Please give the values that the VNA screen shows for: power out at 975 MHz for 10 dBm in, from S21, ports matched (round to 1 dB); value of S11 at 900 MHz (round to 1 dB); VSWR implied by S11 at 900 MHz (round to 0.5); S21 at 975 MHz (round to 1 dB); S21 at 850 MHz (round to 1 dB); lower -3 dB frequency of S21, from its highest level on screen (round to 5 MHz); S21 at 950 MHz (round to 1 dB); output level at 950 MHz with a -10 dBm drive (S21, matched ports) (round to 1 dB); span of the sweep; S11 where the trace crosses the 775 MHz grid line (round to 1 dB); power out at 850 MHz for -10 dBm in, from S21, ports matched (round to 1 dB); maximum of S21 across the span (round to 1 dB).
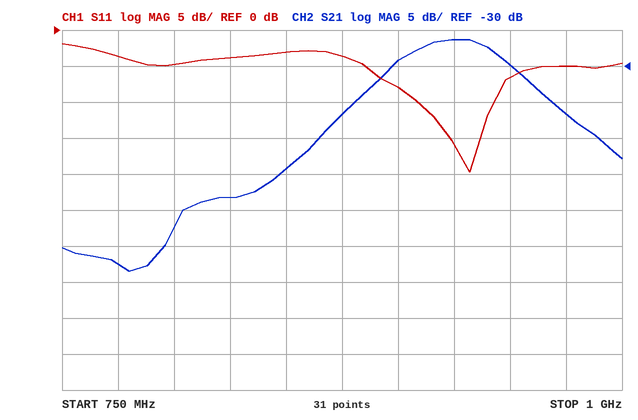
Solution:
-27 dBm
-8 dB
2.5
-37 dB
-44 dB
900 MHz
-30 dB
-40 dBm
250 MHz
-4 dB
-54 dBm
-26 dB
